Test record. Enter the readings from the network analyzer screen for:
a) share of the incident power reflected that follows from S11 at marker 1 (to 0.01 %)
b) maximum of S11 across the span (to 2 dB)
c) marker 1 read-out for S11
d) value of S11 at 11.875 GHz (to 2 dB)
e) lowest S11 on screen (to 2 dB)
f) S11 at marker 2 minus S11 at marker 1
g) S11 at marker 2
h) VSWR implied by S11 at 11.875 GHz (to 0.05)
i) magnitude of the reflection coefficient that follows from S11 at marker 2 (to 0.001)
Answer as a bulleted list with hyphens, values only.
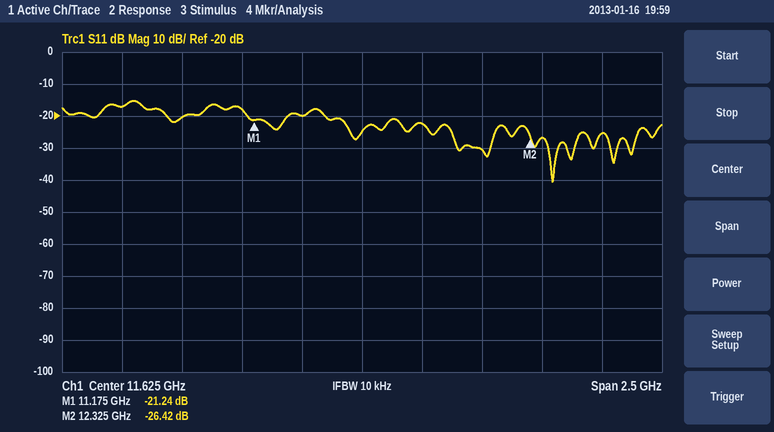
- 0.75 %
- -16 dB
- -21.24 dB
- -22 dB
- -40 dB
- -5.18 dB
- -26.42 dB
- 1.15
- 0.048
